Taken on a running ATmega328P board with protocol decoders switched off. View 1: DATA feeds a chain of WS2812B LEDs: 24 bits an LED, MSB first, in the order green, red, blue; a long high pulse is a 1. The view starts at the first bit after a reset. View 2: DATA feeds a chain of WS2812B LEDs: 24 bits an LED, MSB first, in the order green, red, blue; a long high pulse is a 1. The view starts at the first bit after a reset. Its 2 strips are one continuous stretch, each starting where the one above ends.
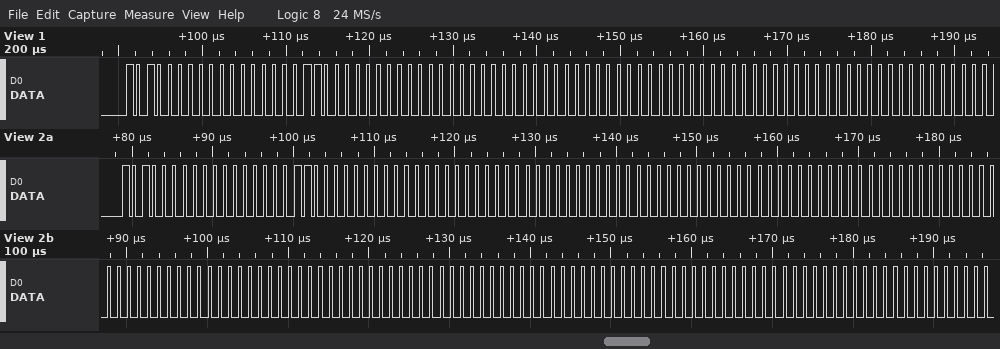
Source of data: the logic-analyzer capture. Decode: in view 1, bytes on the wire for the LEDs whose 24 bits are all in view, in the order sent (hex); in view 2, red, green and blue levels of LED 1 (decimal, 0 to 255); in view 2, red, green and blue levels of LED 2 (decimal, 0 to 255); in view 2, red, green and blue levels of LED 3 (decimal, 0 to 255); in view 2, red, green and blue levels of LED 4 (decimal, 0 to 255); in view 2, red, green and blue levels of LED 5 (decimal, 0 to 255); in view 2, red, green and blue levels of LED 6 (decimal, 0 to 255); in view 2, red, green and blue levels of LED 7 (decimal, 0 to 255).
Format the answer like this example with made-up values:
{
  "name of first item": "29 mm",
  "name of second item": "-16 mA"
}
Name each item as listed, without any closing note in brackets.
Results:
{
  "in view 1, bytes on the wire for the LEDs whose 24 bits are all in view, in the order sent": "A0 00 60 00 00 00 00 00 00",
  "in view 2, red, green and blue levels of LED 1": "0, 160, 96",
  "in view 2, red, green and blue levels of LED 2": "0, 0, 0",
  "in view 2, red, green and blue levels of LED 3": "0, 0, 0",
  "in view 2, red, green and blue levels of LED 4": "0, 0, 0",
  "in view 2, red, green and blue levels of LED 5": "0, 0, 0",
  "in view 2, red, green and blue levels of LED 6": "0, 0, 0",
  "in view 2, red, green and blue levels of LED 7": "0, 0, 0"
}
